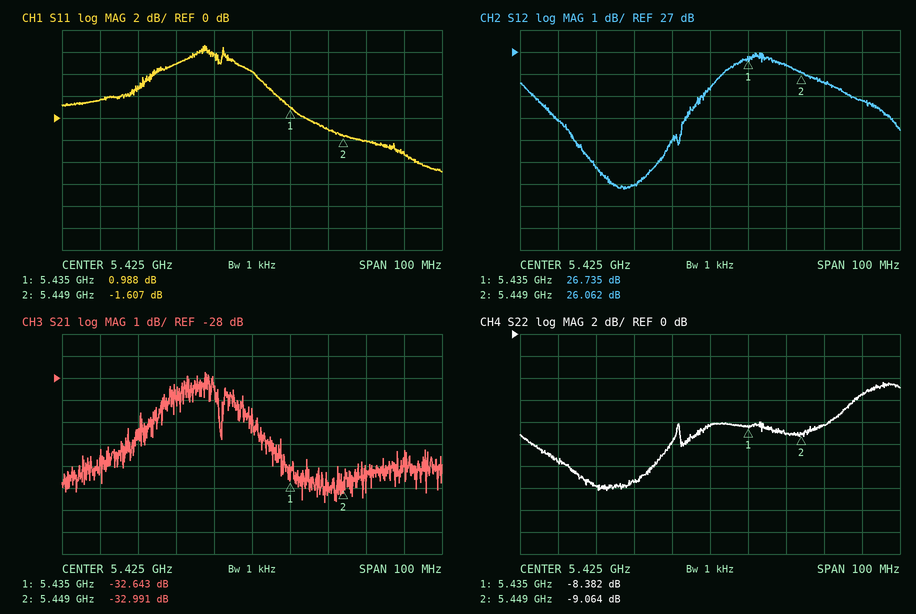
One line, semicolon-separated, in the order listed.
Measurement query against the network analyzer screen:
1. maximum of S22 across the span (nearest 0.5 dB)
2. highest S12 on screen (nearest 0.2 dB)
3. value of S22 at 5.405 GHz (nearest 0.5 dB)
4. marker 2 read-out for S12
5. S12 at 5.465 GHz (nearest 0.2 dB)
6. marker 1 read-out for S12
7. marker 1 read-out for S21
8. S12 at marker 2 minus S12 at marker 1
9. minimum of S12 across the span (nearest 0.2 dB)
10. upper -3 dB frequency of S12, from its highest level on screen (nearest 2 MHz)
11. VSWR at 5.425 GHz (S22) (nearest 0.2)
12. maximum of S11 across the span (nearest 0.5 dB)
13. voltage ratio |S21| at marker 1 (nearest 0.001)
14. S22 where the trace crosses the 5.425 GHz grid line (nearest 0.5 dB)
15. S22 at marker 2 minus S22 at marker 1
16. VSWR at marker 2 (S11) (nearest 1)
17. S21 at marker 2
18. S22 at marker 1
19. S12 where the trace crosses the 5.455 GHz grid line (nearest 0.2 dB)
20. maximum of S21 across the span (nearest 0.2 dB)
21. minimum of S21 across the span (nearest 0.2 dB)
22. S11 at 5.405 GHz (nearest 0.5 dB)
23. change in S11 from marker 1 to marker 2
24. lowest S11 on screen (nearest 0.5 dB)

-4.5 dB; 27.0 dB; -13.5 dB; 26.062 dB; 24.8 dB; 26.735 dB; -32.643 dB; -0.673 dB; 20.8 dB; 5.472 GHz; 2.2; 6.5 dB; 0.023; -8.5 dB; -0.682 dB; 11; -32.991 dB; -8.382 dB; 25.6 dB; -27.8 dB; -33.6 dB; 5.0 dB; -2.595 dB; -5.0 dB
